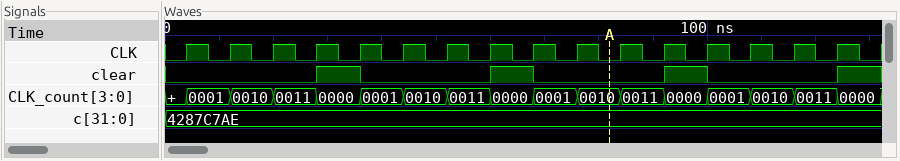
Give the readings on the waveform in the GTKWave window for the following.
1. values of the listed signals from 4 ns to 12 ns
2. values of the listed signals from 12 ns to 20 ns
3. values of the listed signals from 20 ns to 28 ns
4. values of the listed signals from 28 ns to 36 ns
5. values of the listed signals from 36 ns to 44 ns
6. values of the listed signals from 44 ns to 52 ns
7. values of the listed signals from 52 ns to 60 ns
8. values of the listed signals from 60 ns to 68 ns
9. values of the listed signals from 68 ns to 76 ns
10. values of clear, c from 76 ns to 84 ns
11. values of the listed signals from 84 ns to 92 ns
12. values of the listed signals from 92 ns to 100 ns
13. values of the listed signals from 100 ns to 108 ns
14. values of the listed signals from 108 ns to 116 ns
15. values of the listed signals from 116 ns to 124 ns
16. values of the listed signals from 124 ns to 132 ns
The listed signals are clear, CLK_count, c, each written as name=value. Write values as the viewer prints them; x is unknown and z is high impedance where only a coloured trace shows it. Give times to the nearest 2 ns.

clear=0, CLK_count=0001, c=4287C7AE
clear=0, CLK_count=0010, c=4287C7AE
clear=0, CLK_count=0011, c=4287C7AE
clear=1, CLK_count=0000, c=4287C7AE
clear=0, CLK_count=0001, c=4287C7AE
clear=0, CLK_count=0010, c=4287C7AE
clear=0, CLK_count=0011, c=4287C7AE
clear=1, CLK_count=0000, c=4287C7AE
clear=0, CLK_count=0001, c=4287C7AE
clear=0, c=4287C7AE
clear=0, CLK_count=0011, c=4287C7AE
clear=1, CLK_count=0000, c=4287C7AE
clear=0, CLK_count=0001, c=4287C7AE
clear=0, CLK_count=0010, c=4287C7AE
clear=0, CLK_count=0011, c=4287C7AE
clear=1, CLK_count=0000, c=4287C7AE
